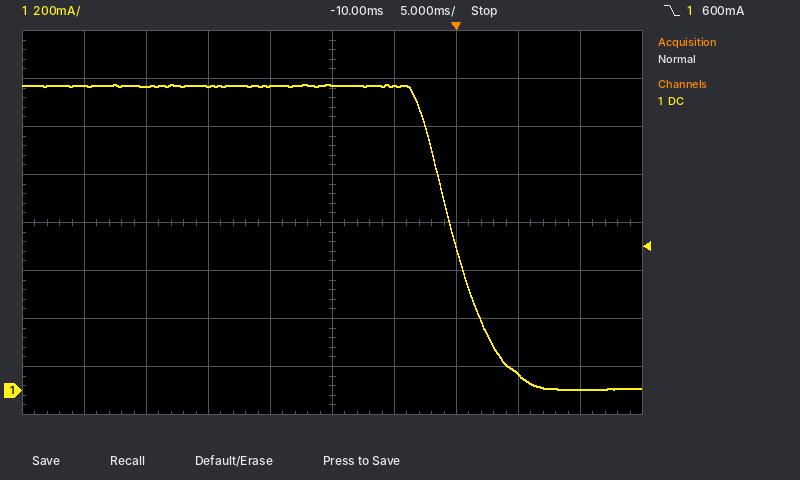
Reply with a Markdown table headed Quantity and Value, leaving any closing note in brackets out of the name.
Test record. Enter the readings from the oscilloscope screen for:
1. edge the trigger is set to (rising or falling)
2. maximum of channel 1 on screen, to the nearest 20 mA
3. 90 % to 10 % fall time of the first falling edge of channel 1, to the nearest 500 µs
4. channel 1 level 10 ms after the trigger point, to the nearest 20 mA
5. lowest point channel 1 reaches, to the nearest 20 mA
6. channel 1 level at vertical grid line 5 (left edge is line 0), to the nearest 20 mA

| Quantity | Value |
|---|---|
| edge the trigger is set to | falling |
| maximum of channel 1 on screen, to the nearest 20 mA | 1.28 A |
| 90 % to 10 % fall time of the first falling edge of channel 1, to the nearest 500 µs | 6.5 ms |
| channel 1 level 10 ms after the trigger point, to the nearest 20 mA | 0 mA |
| lowest point channel 1 reaches, to the nearest 20 mA | 0 mA |
| channel 1 level at vertical grid line 5 (left edge is line 0), to the nearest 20 mA | 1.28 A |
